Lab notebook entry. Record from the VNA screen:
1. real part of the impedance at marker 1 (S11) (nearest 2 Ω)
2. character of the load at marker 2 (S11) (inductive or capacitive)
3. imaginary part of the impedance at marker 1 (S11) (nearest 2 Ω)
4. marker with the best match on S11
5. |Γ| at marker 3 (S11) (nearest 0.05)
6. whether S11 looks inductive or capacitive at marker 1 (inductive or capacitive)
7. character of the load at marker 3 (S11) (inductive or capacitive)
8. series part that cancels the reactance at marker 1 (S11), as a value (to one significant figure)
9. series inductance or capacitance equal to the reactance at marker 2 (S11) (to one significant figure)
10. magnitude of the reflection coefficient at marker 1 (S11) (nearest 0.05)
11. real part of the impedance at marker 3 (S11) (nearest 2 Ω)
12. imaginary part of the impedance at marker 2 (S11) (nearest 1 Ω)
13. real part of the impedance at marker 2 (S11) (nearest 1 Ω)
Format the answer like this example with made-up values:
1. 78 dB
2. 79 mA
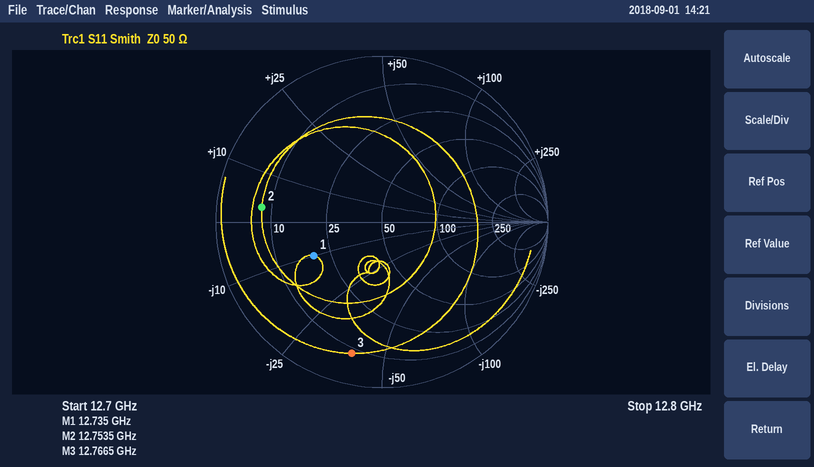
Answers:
1. 20 Ω
2. inductive
3. -10 Ω
4. marker 1
5. 0.80
6. capacitive
7. capacitive
8. 100 pH
9. 40 pH
10. 0.45
11. 8 Ω
12. +3 Ω
13. 8 Ω
